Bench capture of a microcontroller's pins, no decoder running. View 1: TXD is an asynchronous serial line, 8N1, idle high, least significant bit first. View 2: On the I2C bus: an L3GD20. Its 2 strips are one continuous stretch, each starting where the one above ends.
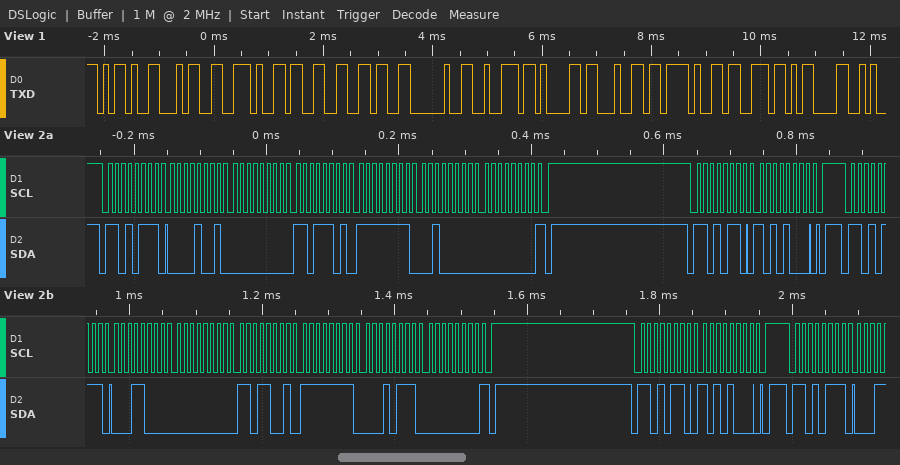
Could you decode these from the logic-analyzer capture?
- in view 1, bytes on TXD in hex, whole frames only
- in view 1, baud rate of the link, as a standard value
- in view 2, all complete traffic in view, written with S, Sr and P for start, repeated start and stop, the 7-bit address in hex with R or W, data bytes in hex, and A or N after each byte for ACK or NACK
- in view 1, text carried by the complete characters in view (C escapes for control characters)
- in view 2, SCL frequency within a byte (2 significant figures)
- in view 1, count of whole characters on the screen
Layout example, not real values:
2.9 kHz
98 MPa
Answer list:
0x2D 0x34 0x2E 0x33 0x36 0x20 0x72 0x61 0x64 0x2F 0x73 0x0D
9600 baud
S 6BR A 09 A 00 A DD A FF A 20 A 00 N P S 6BW A A8 A P S 6BR A 18 A 00 A D9 A FF A 17 A 00 N P S 6BW A A8 A P S 6BR A
"-4.36 rad/s\r"
100 kHz
12
